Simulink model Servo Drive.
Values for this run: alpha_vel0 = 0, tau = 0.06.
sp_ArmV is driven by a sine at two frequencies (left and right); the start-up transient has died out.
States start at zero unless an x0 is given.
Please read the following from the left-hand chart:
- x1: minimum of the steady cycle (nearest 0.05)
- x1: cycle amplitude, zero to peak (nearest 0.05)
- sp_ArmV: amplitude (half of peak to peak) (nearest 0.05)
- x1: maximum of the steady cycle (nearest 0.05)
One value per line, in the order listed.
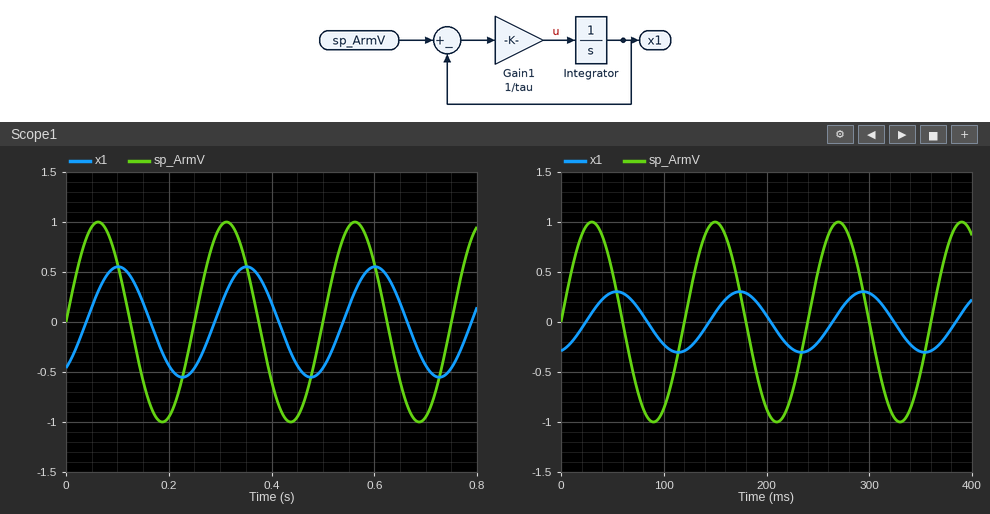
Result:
-0.55
0.55
1.00
0.55
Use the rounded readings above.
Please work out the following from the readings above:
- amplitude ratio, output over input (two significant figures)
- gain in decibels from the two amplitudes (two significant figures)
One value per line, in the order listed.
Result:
0.55
-5.2 dB
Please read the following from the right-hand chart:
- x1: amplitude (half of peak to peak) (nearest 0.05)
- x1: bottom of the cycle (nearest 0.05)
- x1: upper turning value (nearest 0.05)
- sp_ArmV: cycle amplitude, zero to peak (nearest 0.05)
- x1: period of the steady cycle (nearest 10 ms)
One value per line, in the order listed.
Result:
0.30
-0.30
0.30
1.00
120 ms
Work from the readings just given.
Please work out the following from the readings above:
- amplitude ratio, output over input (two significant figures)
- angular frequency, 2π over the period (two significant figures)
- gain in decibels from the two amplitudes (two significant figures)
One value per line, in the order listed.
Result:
0.30
0.052 rad/ms
-10 dB
